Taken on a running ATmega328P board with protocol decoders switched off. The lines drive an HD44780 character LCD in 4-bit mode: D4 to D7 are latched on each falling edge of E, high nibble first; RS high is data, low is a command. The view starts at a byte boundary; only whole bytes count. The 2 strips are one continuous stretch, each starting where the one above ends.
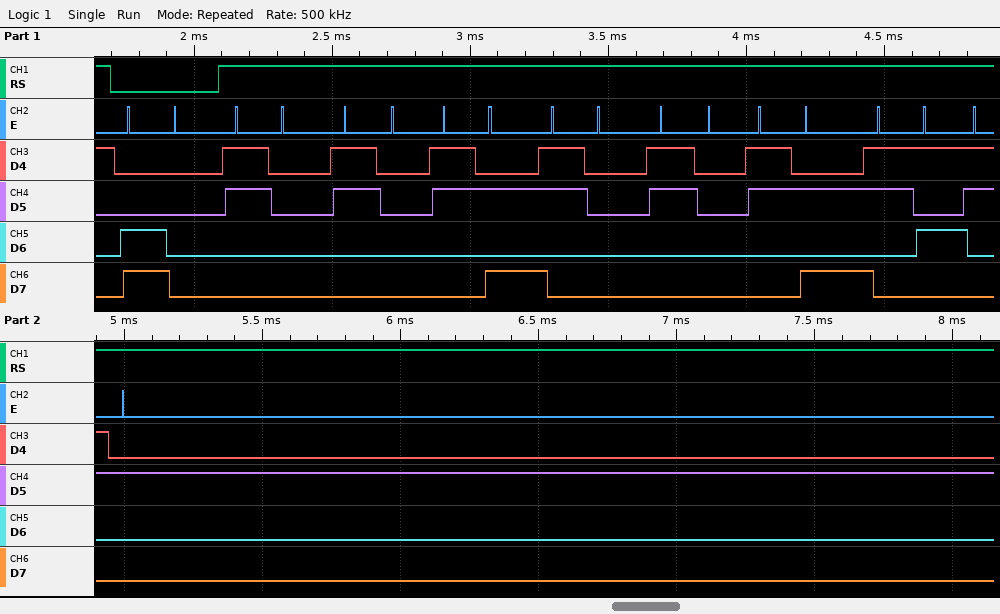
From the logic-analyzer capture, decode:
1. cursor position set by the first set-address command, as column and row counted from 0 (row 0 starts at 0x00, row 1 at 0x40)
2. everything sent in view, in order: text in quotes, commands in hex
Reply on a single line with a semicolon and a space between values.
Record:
column 0, row 1; 0xC0 "00:00:52"
